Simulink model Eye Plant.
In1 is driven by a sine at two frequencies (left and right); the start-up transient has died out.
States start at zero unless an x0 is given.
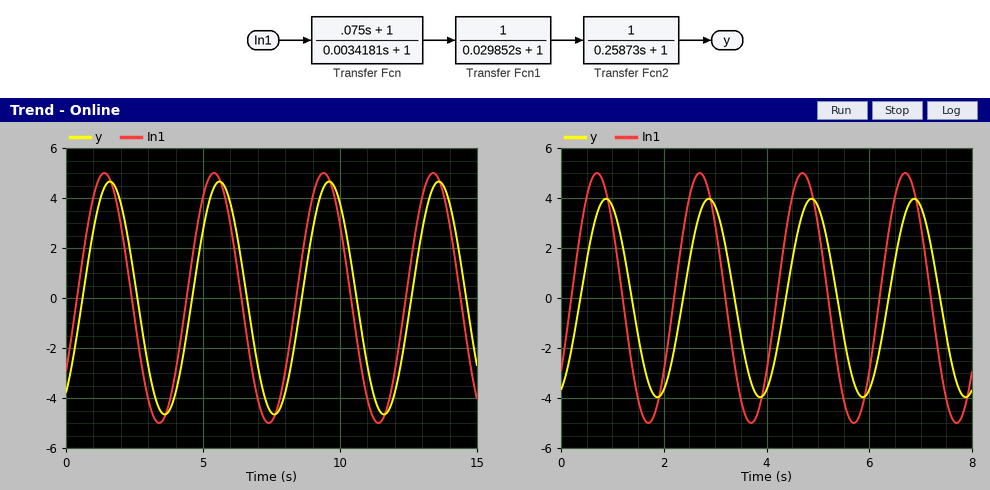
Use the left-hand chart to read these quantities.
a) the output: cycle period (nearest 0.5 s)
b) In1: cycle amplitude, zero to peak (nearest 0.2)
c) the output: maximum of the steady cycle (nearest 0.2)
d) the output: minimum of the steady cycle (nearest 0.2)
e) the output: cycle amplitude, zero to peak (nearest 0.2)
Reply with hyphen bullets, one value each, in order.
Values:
- 4.0 s
- 5.0
- 4.6
- -4.6
- 4.6
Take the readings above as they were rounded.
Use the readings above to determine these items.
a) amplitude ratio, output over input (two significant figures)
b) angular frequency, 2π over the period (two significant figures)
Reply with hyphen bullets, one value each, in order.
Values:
- 0.92
- 1.6 rad/s
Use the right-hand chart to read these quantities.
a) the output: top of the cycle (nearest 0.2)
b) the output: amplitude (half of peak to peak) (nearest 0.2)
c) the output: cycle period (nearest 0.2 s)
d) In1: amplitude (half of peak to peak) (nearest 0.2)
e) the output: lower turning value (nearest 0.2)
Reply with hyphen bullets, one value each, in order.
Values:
- 4.0
- 4.0
- 2.0 s
- 5.0
- -4.0
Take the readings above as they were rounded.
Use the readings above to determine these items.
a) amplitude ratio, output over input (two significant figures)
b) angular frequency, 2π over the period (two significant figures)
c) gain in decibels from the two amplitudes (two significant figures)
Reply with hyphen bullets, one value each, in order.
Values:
- 0.80
- 3.1 rad/s
- -1.9 dB
